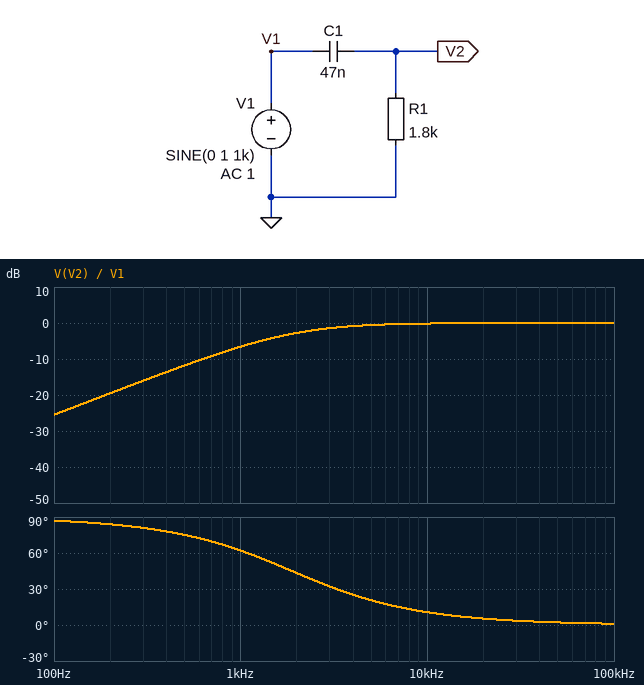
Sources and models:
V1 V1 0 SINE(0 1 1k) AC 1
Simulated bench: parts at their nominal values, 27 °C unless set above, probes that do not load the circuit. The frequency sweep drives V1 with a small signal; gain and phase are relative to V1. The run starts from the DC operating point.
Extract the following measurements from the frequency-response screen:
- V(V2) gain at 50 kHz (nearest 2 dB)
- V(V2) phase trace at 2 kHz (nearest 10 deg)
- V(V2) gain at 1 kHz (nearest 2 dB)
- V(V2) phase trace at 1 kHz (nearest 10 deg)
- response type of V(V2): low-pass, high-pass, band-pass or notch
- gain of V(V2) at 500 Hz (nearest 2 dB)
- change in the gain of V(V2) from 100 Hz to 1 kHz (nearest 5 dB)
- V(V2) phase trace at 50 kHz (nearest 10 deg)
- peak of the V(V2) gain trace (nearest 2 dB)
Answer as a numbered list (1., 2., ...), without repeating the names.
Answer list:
1. 0 dB
2. 40 deg
3. -6 dB
4. 60 deg
5. high-pass
6. -12 dB
7. 20 dB
8. 0 deg
9. 0 dB
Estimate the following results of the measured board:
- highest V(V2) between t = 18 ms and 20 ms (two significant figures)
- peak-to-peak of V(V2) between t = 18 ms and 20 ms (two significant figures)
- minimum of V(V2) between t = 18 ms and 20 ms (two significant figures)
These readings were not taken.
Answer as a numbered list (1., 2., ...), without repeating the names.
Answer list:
1. 470 mV
2. 940 mV
3. -470 mV
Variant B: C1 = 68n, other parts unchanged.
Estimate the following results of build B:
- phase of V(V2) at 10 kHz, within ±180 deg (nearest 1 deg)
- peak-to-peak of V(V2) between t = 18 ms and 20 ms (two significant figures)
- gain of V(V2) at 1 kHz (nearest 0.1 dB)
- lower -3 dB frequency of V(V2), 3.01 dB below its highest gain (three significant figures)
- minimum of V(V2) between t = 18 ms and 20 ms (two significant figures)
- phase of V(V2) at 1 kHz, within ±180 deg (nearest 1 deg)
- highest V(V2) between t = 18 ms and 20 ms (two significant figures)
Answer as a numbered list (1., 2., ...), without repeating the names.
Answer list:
1. 7 deg
2. 1.2 V
3. -4.3 dB
4. 1.30 kHz
5. -610 mV
6. 52 deg
7. 610 mV
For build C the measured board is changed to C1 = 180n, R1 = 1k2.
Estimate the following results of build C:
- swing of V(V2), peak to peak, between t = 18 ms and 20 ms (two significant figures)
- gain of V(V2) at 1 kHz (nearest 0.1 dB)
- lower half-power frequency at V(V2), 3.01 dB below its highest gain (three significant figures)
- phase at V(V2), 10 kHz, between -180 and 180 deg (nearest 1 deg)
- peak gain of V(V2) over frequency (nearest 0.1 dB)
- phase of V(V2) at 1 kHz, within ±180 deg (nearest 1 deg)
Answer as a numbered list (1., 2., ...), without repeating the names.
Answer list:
1. 1.6 V
2. -1.9 dB
3. 737 Hz
4. 4 deg
5. 0 dB
6. 36 deg
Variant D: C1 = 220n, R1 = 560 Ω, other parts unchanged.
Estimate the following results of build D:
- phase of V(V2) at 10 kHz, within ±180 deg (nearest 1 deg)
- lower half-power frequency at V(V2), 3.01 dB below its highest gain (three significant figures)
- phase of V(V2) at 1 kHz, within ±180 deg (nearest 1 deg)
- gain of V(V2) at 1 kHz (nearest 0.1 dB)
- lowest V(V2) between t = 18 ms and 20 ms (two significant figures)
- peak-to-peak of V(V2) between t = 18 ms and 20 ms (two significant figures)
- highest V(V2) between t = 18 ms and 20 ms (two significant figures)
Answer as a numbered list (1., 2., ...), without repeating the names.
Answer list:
1. 7 deg
2. 1.29 kHz
3. 52 deg
4. -4.3 dB
5. -610 mV
6. 1.2 V
7. 610 mV
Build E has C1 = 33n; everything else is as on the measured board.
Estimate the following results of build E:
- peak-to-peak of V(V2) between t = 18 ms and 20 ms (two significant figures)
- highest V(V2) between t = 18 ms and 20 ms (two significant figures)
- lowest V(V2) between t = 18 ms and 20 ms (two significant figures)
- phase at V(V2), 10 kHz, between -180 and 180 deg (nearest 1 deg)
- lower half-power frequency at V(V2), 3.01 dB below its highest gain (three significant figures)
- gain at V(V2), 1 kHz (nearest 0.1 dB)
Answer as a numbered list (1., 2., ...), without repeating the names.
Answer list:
1. 700 mV
2. 350 mV
3. -350 mV
4. 15 deg
5. 2.68 kHz
6. -9.1 dB
